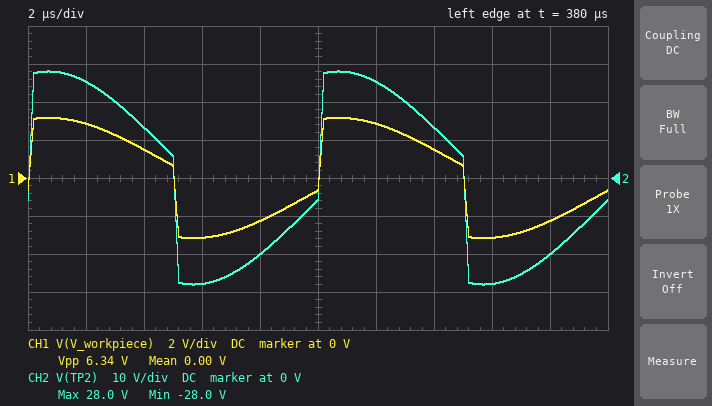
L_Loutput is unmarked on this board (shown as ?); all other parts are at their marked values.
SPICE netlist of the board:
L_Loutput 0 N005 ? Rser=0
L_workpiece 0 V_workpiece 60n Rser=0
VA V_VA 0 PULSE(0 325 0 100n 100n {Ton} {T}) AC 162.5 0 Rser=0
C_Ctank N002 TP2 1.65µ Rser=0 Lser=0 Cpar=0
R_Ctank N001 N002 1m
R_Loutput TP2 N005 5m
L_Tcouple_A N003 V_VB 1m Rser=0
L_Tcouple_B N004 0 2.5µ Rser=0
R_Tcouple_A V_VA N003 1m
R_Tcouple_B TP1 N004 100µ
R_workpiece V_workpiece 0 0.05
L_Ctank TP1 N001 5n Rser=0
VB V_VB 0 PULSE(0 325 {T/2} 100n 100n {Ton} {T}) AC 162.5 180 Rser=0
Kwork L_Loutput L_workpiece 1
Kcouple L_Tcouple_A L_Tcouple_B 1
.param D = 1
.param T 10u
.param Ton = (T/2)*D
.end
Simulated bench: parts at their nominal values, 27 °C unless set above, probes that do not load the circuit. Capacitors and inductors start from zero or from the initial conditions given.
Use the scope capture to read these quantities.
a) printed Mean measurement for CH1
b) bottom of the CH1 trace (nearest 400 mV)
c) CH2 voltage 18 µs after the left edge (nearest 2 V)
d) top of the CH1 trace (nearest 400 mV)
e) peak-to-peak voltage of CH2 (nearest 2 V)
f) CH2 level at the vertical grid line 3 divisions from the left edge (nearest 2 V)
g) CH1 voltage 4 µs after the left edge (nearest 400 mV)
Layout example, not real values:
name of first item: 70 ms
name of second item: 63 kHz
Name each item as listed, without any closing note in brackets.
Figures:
printed Mean measurement for CH1: 0.00 V
bottom of the CH1 trace: -3.2 V
CH2 voltage 18 µs after the left edge: -20 V
top of the CH1 trace: 3.2 V
peak-to-peak voltage of CH2: 56 V
CH2 level at the vertical grid line 3 divisions from the left edge: -28 V
CH1 voltage 4 µs after the left edge: 1.6 V
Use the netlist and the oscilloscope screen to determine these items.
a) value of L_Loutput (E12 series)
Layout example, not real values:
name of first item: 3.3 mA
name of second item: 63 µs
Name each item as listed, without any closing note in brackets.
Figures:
value of L_Loutput: 4.7 µH
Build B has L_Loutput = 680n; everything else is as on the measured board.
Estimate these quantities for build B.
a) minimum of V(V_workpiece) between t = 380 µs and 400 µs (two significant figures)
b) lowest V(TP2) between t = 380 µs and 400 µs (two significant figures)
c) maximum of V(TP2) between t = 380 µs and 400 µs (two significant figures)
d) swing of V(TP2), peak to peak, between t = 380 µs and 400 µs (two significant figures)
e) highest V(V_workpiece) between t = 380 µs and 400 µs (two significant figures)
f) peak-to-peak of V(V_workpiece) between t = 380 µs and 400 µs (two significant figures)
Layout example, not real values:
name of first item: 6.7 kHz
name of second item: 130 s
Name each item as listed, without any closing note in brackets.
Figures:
minimum of V(V_workpiece) between t = 380 µs and 400 µs: -8.5 V
lowest V(TP2) between t = 380 µs and 400 µs: -29 V
maximum of V(TP2) between t = 380 µs and 400 µs: 29 V
swing of V(TP2), peak to peak, between t = 380 µs and 400 µs: 58 V
highest V(V_workpiece) between t = 380 µs and 400 µs: 8.5 V
peak-to-peak of V(V_workpiece) between t = 380 µs and 400 µs: 17 V
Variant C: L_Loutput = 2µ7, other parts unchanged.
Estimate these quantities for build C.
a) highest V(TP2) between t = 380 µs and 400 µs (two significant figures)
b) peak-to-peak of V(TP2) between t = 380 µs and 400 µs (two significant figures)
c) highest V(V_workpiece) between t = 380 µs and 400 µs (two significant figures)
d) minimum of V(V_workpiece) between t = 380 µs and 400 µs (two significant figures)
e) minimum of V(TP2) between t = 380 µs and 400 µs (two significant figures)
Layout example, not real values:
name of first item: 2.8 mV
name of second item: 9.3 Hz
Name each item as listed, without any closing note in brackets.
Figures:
highest V(TP2) between t = 380 µs and 400 µs: 42 V
peak-to-peak of V(TP2) between t = 380 µs and 400 µs: 84 V
highest V(V_workpiece) between t = 380 µs and 400 µs: 6.3 V
minimum of V(V_workpiece) between t = 380 µs and 400 µs: -6.3 V
minimum of V(TP2) between t = 380 µs and 400 µs: -42 V
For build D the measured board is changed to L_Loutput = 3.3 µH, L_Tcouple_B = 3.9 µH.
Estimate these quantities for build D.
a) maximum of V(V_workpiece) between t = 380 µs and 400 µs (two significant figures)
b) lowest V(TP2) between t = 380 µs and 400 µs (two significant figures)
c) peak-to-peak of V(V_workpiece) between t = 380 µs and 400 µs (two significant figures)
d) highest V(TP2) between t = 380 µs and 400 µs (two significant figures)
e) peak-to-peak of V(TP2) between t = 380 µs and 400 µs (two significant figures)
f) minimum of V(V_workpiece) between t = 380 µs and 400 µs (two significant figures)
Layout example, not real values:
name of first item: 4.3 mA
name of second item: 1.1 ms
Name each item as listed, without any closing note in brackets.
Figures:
maximum of V(V_workpiece) between t = 380 µs and 400 µs: 6.0 V
lowest V(TP2) between t = 380 µs and 400 µs: -45 V
peak-to-peak of V(V_workpiece) between t = 380 µs and 400 µs: 12 V
highest V(TP2) between t = 380 µs and 400 µs: 45 V
peak-to-peak of V(TP2) between t = 380 µs and 400 µs: 89 V
minimum of V(V_workpiece) between t = 380 µs and 400 µs: -6.0 V
